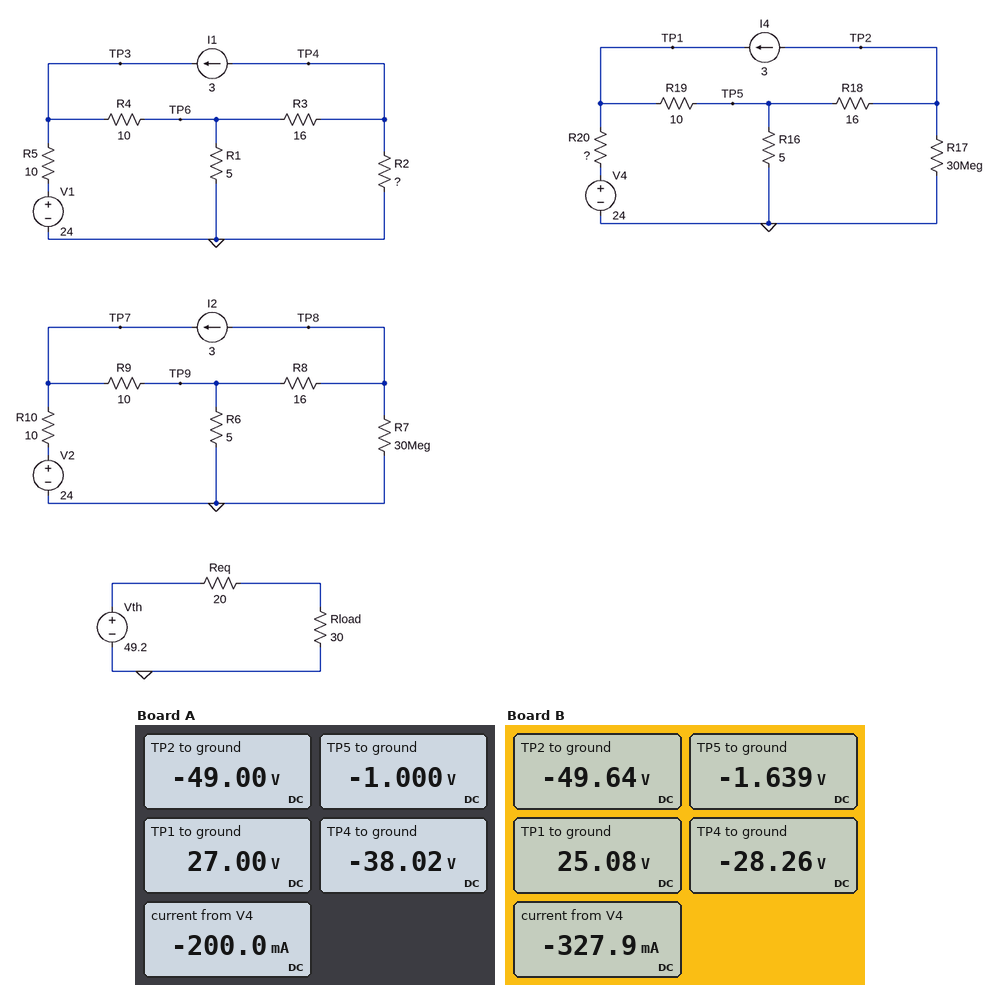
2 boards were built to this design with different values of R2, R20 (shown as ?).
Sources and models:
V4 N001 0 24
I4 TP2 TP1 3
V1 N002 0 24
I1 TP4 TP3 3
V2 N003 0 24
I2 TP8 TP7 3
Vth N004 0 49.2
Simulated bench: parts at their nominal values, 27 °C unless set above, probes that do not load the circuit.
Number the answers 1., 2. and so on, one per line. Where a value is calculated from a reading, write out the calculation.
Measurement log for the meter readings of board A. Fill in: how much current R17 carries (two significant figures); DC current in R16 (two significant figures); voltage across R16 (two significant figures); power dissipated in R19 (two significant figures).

1. (0 V - (-49 V)) / 30 MΩ = 1.6 µA
2. (0 V - (-1 V)) / 5 Ω = 200 mA
3. 0 V - (-1 V) = 1.0 V
4. (27 V - (-1 V))^2 / 10 Ω = 78 W
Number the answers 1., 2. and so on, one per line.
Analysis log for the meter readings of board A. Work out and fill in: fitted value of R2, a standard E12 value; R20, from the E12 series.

1. 68 Ω
2. 15 Ω
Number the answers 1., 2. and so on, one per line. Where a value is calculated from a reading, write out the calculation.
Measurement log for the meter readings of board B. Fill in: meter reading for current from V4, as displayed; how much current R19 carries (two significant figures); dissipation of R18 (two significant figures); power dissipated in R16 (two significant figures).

1. -327.9 mA
2. (25.08 V - (-1.639 V)) / 10 Ω = 2.7 A
3. (-1.639 V - (-49.64 V))^2 / 16 Ω = 140 W
4. (0 V - (-1.639 V))^2 / 5 Ω = 540 mW
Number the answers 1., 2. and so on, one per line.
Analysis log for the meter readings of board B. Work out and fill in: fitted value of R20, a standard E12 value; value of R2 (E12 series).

1. 3.3 Ω
2. 27 Ω
